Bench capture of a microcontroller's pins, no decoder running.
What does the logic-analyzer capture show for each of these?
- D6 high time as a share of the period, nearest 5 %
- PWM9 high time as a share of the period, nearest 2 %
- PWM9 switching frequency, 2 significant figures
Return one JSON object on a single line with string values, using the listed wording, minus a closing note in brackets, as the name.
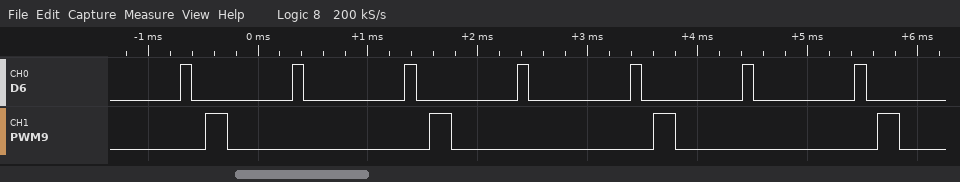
{"D6 high time as a share of the period, nearest 5 %": "10 %", "PWM9 high time as a share of the period, nearest 2 %": "10 %", "PWM9 switching frequency, 2 significant figures": "490 Hz"}
